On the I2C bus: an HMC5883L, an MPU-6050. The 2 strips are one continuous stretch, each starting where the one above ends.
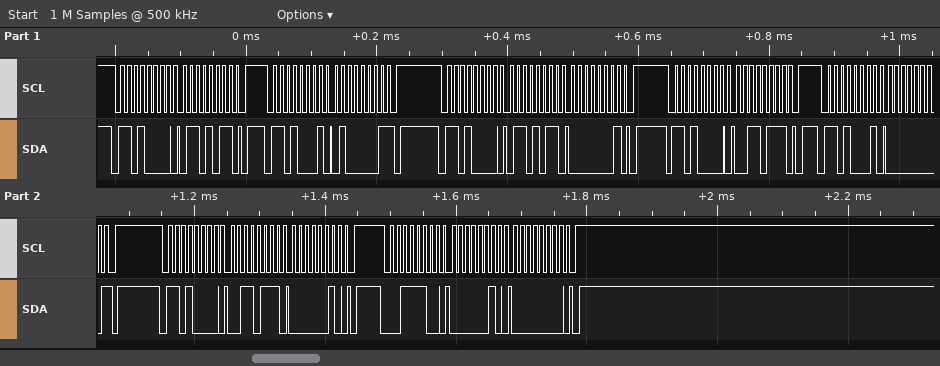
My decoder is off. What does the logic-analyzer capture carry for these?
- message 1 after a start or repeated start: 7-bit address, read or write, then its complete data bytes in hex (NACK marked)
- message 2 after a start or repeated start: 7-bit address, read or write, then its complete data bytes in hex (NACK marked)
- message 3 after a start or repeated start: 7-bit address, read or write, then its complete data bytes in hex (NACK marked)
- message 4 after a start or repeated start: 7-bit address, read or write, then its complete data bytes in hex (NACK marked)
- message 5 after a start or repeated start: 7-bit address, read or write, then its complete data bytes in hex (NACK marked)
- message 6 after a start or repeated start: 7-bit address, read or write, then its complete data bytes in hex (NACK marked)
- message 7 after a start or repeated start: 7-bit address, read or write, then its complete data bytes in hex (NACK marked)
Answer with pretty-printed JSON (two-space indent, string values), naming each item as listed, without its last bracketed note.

{
  "message 1 after a start or repeated start: 7-bit address, read or write, then its complete data bytes in hex": "0x68 write: 6B",
  "message 2 after a start or repeated start: 7-bit address, read or write, then its complete data bytes in hex": "0x68 read: 41 NACK",
  "message 3 after a start or repeated start: 7-bit address, read or write, then its complete data bytes in hex": "0x68 write: 6B 01",
  "message 4 after a start or repeated start: 7-bit address, read or write, then its complete data bytes in hex": "0x68 write: 37",
  "message 5 after a start or repeated start: 7-bit address, read or write, then its complete data bytes in hex": "0x68 read: 00 NACK",
  "message 6 after a start or repeated start: 7-bit address, read or write, then its complete data bytes in hex": "0x68 write: 37 02",
  "message 7 after a start or repeated start: 7-bit address, read or write, then its complete data bytes in hex": "0x1E write: 02 00"
}
